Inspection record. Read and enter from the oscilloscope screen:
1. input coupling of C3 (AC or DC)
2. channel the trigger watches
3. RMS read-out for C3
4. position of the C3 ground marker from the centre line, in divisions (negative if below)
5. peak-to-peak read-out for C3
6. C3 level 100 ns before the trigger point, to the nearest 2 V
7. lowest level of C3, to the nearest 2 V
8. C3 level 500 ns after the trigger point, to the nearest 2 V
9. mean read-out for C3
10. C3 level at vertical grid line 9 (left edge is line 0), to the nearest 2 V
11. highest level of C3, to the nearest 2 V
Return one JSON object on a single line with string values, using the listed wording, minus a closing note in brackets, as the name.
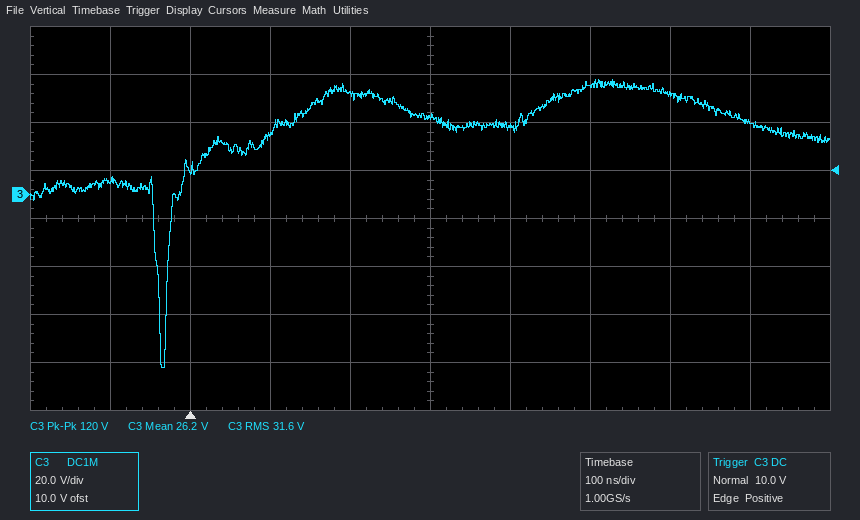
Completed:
{"input coupling of C3": "DC", "channel the trigger watches": "C3", "RMS read-out for C3": "31.6 V", "position of the C3 ground marker from the centre line, in divisions": "+0.5 div", "peak-to-peak read-out for C3": "120 V", "C3 level 100 ns before the trigger point, to the nearest 2 V": "6 V", "lowest level of C3, to the nearest 2 V": "-72 V", "C3 level 500 ns after the trigger point, to the nearest 2 V": "46 V", "mean read-out for C3": "26.2 V", "C3 level at vertical grid line 9 (left edge is line 0), to the nearest 2 V": "30 V", "highest level of C3, to the nearest 2 V": "48 V"}
